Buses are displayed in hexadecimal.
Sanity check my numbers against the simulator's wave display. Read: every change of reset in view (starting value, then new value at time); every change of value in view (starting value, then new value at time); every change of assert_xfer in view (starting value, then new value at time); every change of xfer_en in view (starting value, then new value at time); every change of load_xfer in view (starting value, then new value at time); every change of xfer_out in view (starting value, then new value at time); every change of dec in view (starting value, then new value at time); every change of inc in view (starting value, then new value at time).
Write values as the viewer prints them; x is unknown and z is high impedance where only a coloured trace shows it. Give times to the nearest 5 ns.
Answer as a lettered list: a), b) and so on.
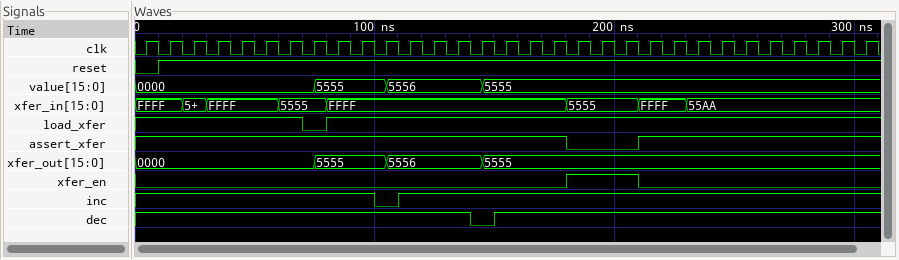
a) 0, 1 at 10 ns
b) 0000, 5555 at 75 ns, 5556 at 105 ns, 5555 at 145 ns
c) 1, 0 at 180 ns, 1 at 210 ns
d) 0, 1 at 180 ns, 0 at 210 ns
e) 1, 0 at 70 ns, 1 at 80 ns
f) 0000, 5555 at 75 ns, 5556 at 105 ns, 5555 at 145 ns
g) 1, 0 at 140 ns, 1 at 150 ns
h) 1, 0 at 100 ns, 1 at 110 ns
